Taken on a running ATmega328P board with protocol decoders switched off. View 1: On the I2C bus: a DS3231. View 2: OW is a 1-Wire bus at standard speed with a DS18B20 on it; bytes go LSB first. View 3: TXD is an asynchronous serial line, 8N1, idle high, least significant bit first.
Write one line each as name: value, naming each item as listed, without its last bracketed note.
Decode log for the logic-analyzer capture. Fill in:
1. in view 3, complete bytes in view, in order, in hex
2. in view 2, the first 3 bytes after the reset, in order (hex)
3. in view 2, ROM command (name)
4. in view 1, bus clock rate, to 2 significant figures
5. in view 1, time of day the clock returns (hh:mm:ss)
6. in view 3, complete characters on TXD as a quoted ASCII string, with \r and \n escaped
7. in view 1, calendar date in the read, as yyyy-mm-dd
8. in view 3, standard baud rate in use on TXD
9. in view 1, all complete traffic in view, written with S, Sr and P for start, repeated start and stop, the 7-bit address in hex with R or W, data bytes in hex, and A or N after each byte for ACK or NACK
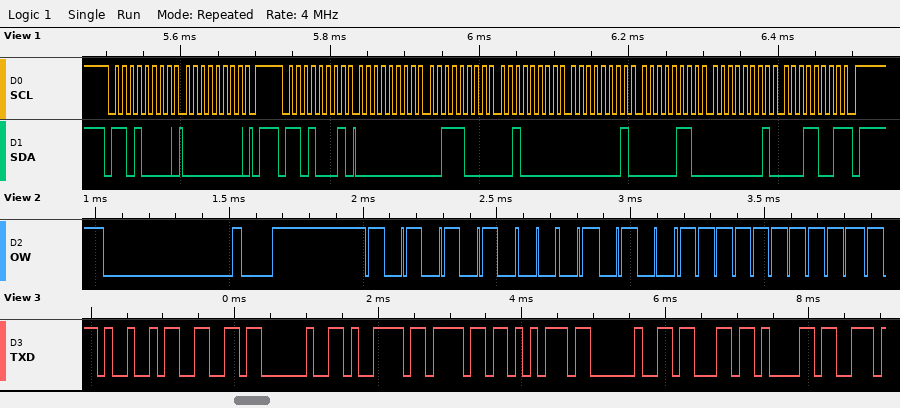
in view 3, complete bytes in view, in order, in hex: 49 66 20 79 6F 75 20 63 61
in view 2, the first 3 bytes after the reset, in order: 55 28 FF
in view 2, ROM command: Match ROM
in view 1, bus clock rate, to 2 significant figures: 100 kHz
in view 1, time of day the clock returns: 20:38:00
in view 3, complete characters on TXD as a quoted ASCII string, with \r and \n escaped: "If you ca"
in view 1, calendar date in the read, as yyyy-mm-dd: 2019-01-06
in view 3, standard baud rate in use on TXD: 9600 baud
in view 1, all complete traffic in view, written with S, Sr and P for start, repeated start and stop, the 7-bit address in hex with R or W, data bytes in hex, and A or N after each byte for ACK or NACK: S 68W A 00 A P S 68R A 00 A 38 A 20 A 01 A 06 A 01 A 19 N P
